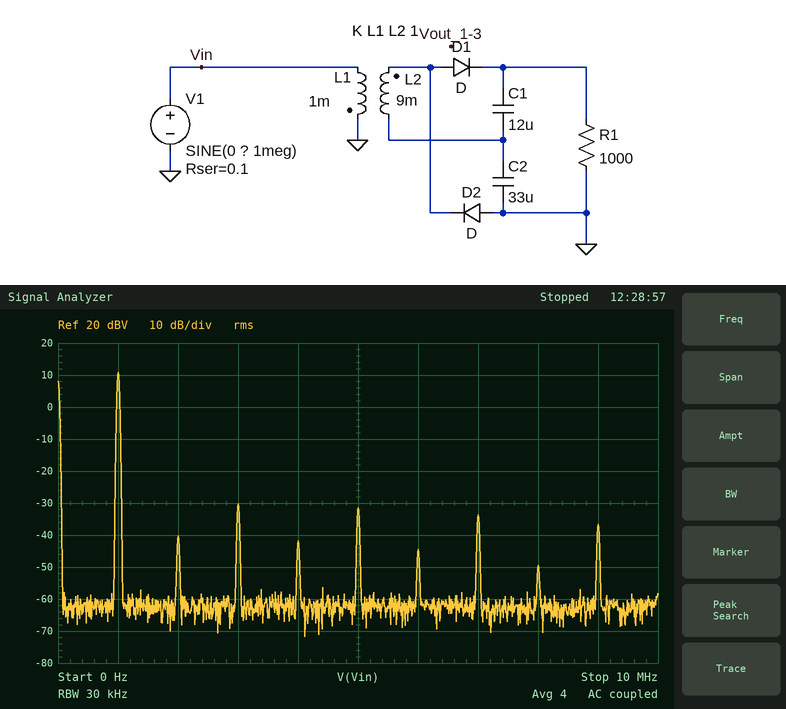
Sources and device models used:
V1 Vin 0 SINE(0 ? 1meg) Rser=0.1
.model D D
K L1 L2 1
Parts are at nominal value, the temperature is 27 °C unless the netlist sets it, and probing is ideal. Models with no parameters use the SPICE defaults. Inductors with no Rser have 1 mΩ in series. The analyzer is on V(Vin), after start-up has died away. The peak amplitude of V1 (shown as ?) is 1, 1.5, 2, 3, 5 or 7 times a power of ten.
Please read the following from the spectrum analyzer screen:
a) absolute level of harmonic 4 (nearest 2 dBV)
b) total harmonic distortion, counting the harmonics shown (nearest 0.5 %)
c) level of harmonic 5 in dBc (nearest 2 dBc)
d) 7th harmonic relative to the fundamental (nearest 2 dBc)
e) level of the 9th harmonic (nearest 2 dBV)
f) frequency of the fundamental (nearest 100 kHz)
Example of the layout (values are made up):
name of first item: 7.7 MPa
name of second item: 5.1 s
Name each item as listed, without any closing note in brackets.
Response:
absolute level of harmonic 4: -42 dBV
total harmonic distortion, counting the harmonics shown: 1.5 %
level of harmonic 5 in dBc: -42 dBc
7th harmonic relative to the fundamental: -44 dBc
level of the 9th harmonic: -36 dBV
frequency of the fundamental: 1.0 MHz
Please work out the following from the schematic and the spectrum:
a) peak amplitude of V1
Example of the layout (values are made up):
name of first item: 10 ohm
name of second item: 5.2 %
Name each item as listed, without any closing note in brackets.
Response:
peak amplitude of V1: 5 V
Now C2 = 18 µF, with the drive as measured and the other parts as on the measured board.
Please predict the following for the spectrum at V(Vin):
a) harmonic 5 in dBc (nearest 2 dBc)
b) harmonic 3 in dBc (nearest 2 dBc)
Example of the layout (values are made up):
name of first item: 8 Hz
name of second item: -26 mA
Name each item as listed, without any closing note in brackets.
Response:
harmonic 5 in dBc: -44 dBc
harmonic 3 in dBc: -44 dBc
